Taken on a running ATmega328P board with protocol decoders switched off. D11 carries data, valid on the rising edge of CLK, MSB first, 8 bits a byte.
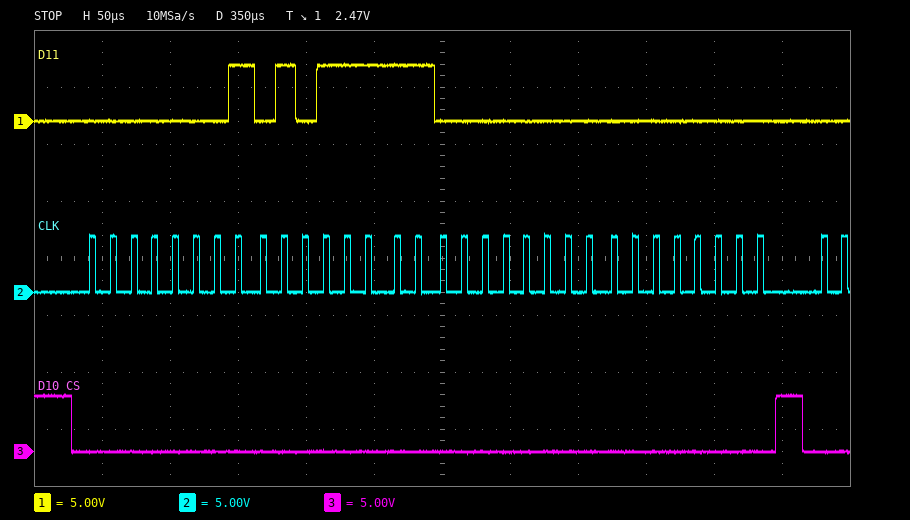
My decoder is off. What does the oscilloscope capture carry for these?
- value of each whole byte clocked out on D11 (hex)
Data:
0x01 0x5F 0x00 0x00
